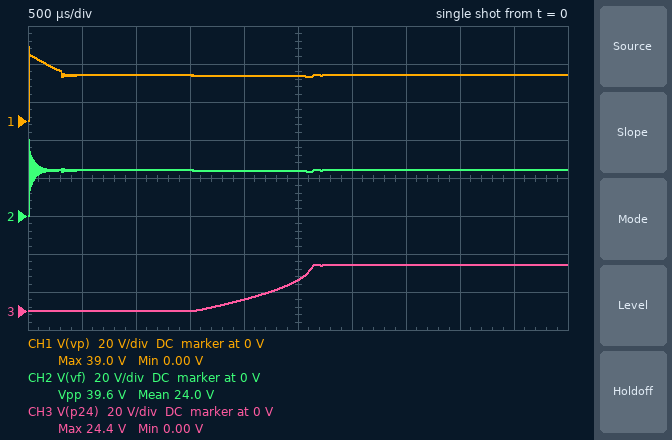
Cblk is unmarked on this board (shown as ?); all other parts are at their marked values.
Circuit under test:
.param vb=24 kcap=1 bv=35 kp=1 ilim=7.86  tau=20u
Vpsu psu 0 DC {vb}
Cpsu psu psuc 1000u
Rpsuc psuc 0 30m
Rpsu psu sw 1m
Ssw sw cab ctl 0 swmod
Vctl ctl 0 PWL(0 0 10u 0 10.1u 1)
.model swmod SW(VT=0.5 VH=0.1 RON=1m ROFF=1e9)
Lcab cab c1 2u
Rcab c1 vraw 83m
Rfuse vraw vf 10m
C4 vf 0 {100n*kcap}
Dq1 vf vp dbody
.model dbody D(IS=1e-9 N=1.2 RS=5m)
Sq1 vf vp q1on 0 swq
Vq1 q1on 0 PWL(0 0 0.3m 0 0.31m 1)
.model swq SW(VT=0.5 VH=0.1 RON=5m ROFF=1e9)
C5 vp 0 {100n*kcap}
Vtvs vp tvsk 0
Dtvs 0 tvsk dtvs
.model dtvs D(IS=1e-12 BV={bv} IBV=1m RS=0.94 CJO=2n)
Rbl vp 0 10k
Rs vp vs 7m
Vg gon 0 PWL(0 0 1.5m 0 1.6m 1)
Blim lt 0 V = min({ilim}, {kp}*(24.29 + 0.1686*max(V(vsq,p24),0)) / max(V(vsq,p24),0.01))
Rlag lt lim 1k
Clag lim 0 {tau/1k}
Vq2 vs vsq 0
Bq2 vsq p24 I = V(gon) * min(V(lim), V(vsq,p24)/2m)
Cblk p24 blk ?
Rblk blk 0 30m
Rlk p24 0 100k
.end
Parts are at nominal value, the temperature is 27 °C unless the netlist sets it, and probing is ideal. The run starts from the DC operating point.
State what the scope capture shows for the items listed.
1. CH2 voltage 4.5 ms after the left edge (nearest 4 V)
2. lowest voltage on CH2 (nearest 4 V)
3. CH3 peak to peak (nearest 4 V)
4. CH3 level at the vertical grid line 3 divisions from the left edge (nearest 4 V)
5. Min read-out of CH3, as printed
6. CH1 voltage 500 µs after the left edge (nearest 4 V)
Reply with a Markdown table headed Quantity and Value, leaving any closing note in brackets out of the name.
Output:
| Quantity | Value |
|---|---|
| CH2 voltage 4.5 ms after the left edge | 24 V |
| lowest voltage on CH2 | 0 V |
| CH3 peak to peak | 24 V |
| CH3 level at the vertical grid line 3 divisions from the left edge | 0 V |
| Min read-out of CH3, as printed | 0.00 V |
| CH1 voltage 500 µs after the left edge | 24 V |
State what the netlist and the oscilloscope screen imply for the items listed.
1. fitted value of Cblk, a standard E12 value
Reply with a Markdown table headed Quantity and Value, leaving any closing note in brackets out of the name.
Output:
| Quantity | Value |
|---|---|
| fitted value of Cblk, a standard E12 value | 100 µF |
